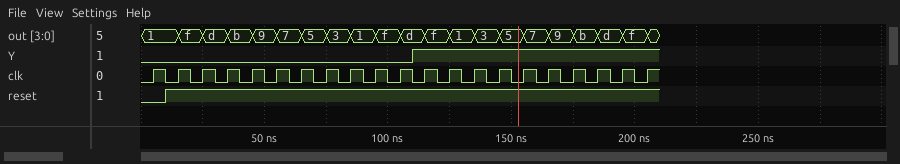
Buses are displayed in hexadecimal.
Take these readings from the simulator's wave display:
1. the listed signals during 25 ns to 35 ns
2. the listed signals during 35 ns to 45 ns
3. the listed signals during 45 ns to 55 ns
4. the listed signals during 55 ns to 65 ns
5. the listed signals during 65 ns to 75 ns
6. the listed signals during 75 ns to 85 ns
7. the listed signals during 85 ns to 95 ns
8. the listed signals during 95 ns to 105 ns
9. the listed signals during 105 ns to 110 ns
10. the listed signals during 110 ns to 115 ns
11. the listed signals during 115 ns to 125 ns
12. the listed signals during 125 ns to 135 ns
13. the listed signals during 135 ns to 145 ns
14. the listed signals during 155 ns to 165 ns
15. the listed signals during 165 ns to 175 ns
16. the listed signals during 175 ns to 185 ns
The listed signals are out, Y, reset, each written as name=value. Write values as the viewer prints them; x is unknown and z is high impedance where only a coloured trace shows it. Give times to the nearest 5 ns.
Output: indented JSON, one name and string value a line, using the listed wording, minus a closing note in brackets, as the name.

{
  "the listed signals during 25 ns to 35 ns": "out=d, Y=0, reset=1",
  "the listed signals during 35 ns to 45 ns": "out=b, Y=0, reset=1",
  "the listed signals during 45 ns to 55 ns": "out=9, Y=0, reset=1",
  "the listed signals during 55 ns to 65 ns": "out=7, Y=0, reset=1",
  "the listed signals during 65 ns to 75 ns": "out=5, Y=0, reset=1",
  "the listed signals during 75 ns to 85 ns": "out=3, Y=0, reset=1",
  "the listed signals during 85 ns to 95 ns": "out=1, Y=0, reset=1",
  "the listed signals during 95 ns to 105 ns": "out=f, Y=0, reset=1",
  "the listed signals during 105 ns to 110 ns": "out=d, Y=0, reset=1",
  "the listed signals during 110 ns to 115 ns": "out=d, Y=1, reset=1",
  "the listed signals during 115 ns to 125 ns": "out=f, Y=1, reset=1",
  "the listed signals during 125 ns to 135 ns": "out=1, Y=1, reset=1",
  "the listed signals during 135 ns to 145 ns": "out=3, Y=1, reset=1",
  "the listed signals during 155 ns to 165 ns": "out=7, Y=1, reset=1",
  "the listed signals during 165 ns to 175 ns": "out=9, Y=1, reset=1",
  "the listed signals during 175 ns to 185 ns": "out=b, Y=1, reset=1"
}
